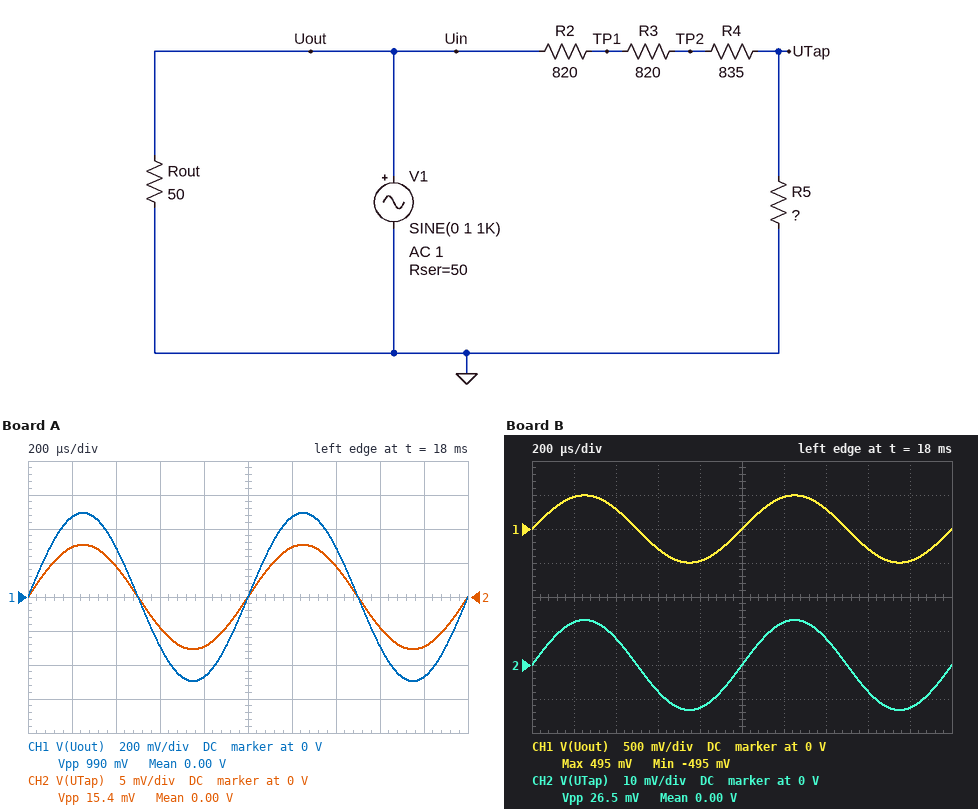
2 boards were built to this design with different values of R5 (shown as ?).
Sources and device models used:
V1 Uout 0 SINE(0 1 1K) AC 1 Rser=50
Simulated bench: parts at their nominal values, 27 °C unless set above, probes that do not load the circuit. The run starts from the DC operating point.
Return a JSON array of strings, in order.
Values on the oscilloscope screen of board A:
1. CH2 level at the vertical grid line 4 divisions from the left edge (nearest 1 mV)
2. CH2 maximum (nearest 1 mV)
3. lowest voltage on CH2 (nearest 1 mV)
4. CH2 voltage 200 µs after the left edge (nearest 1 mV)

["-7 mV", "8 mV", "-8 mV", "7 mV"]
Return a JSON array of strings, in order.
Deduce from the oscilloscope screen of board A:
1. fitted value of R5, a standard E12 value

["39 Ω"]
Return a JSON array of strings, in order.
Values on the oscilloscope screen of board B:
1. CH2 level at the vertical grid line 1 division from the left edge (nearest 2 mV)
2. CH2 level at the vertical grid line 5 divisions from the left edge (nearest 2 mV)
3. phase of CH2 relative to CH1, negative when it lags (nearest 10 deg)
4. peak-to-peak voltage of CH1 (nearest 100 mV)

["12 mV", "0 V", "0 deg", "1.0 V"]
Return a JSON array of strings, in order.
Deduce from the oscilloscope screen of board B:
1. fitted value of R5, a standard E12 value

["68 Ω"]
